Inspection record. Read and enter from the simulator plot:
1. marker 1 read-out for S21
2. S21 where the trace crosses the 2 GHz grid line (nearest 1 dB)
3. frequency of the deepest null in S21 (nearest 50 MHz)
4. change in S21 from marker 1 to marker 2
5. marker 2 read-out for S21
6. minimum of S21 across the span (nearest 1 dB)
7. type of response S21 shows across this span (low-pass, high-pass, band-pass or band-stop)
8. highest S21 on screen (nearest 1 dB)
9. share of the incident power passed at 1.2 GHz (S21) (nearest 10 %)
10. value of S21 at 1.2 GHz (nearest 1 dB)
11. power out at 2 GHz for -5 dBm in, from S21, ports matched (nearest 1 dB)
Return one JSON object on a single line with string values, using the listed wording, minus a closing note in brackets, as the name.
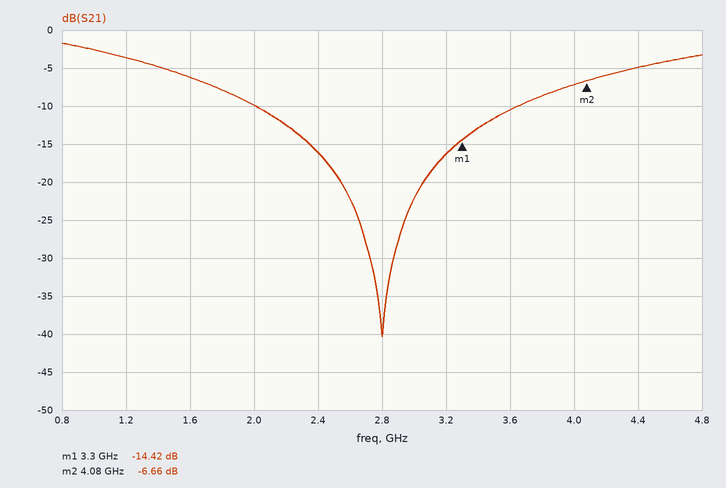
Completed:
{"marker 1 read-out for S21": "-14.42 dB", "S21 where the trace crosses the 2 GHz grid line": "-10 dB", "frequency of the deepest null in S21": "2.80 GHz", "change in S21 from marker 1 to marker 2": "7.76 dB", "marker 2 read-out for S21": "-6.66 dB", "minimum of S21 across the span": "-40 dB", "type of response S21 shows across this span": "band-stop", "highest S21 on screen": "-2 dB", "share of the incident power passed at 1.2 GHz (S21)": "40 %", "value of S21 at 1.2 GHz": "-4 dB", "power out at 2 GHz for -5 dBm in, from S21, ports matched": "-15 dBm"}
